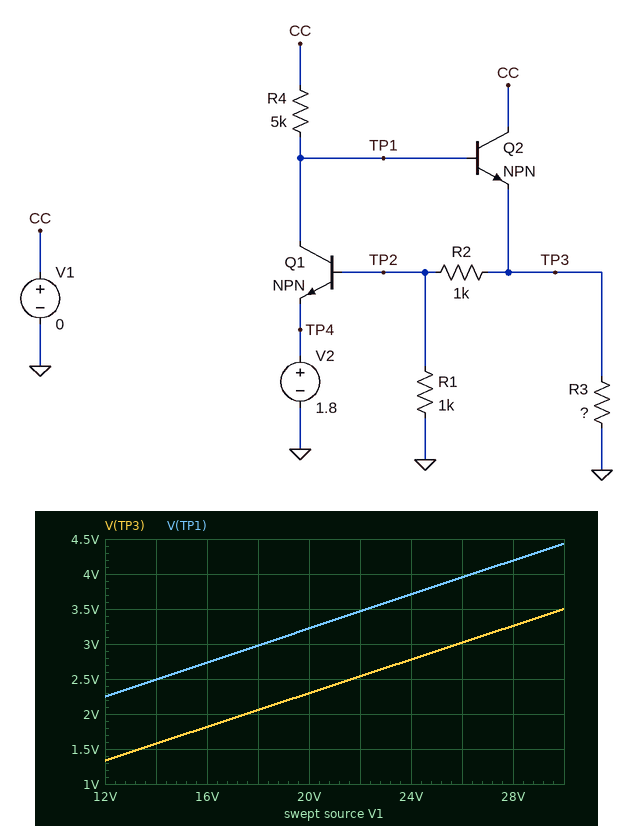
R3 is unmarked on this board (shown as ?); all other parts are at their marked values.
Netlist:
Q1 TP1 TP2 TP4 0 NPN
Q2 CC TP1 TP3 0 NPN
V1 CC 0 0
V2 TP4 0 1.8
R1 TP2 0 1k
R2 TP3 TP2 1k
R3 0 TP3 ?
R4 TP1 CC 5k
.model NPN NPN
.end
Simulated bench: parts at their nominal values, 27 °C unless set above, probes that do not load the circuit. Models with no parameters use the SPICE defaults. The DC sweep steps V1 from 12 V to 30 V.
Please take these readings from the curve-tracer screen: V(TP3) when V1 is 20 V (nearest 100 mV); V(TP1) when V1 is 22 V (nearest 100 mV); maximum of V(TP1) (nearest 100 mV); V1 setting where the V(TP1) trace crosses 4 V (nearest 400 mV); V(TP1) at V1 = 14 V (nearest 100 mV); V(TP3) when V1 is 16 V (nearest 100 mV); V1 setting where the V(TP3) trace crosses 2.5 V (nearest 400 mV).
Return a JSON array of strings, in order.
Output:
["2.3 V", "3.5 V", "4.4 V", "26.4 V", "2.5 V", "1.8 V", "21.6 V"]
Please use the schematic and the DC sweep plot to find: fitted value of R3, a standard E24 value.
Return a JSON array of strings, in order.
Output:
["6.8 Ω"]
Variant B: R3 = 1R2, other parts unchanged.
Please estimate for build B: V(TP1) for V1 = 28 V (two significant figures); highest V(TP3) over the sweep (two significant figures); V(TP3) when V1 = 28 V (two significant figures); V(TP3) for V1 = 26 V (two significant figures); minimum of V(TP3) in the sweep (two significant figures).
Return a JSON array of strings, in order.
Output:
["1.6 V", "690 mV", "640 mV", "590 mV", "260 mV"]
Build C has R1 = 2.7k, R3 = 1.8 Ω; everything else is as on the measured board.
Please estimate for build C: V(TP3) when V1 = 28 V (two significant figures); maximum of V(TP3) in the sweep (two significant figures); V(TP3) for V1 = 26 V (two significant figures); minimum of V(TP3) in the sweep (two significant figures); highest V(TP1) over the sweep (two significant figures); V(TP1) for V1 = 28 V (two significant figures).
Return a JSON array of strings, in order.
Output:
["950 mV", "1.0 V", "880 mV", "390 mV", "2.0 V", "1.9 V"]
